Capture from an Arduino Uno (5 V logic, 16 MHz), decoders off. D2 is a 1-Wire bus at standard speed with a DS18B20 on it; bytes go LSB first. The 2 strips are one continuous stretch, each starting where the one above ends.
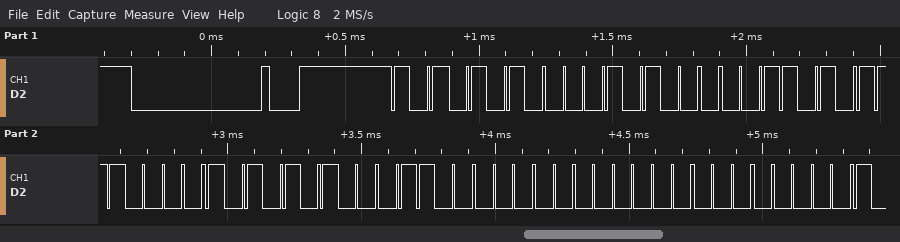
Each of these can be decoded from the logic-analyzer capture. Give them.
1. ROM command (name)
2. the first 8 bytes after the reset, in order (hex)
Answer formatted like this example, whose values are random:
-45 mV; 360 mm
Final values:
Match ROM; 55 28 58 87 2A 06 00 00
